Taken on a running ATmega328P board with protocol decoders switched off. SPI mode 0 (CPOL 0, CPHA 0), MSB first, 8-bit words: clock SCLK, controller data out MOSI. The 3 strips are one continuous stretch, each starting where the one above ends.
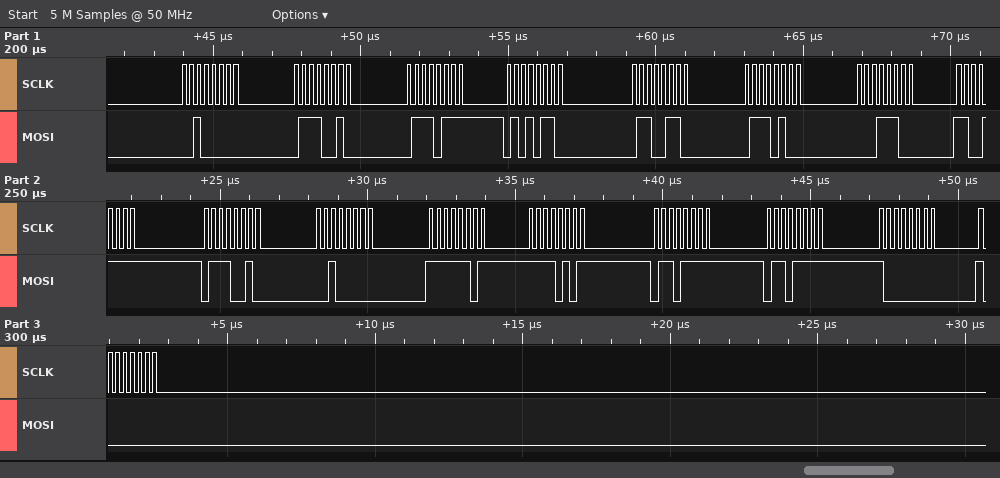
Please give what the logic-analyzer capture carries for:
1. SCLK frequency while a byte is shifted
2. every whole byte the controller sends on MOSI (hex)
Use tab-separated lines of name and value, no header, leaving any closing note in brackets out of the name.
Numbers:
SCLK frequency while a byte is shifted	4 MHz
every whole byte the controller sends on MOSI	20 72 77 56 66 74 1C CF 72 20 FD F5 6F 6F 80 80
